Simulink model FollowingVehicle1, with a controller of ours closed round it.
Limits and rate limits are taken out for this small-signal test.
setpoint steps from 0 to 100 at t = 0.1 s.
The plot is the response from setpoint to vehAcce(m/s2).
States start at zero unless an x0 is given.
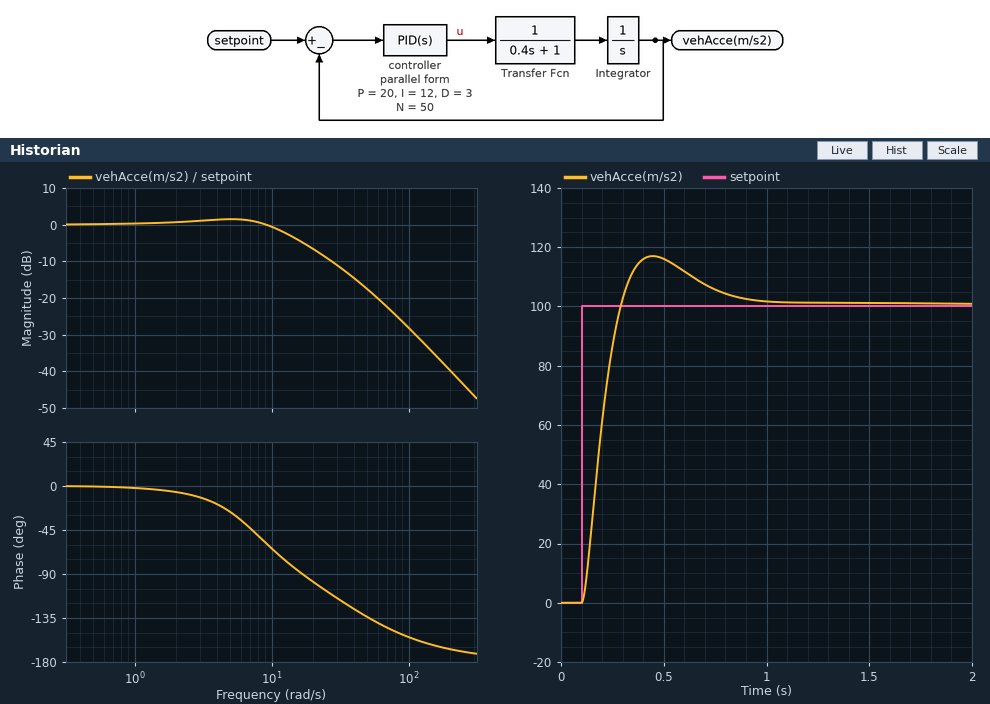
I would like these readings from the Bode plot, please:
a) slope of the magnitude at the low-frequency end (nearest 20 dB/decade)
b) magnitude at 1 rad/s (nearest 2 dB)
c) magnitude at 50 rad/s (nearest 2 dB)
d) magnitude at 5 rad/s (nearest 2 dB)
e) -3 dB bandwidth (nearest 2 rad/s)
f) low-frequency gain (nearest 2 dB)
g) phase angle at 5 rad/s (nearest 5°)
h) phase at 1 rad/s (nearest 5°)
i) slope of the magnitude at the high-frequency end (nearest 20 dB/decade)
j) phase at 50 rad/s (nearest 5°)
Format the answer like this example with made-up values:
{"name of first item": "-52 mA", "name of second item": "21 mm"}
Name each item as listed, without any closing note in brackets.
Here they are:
{"slope of the magnitude at the low-frequency end": "0 dB/decade", "magnitude at 1 rad/s": "0 dB", "magnitude at 50 rad/s": "-18 dB", "magnitude at 5 rad/s": "2 dB", "-3 dB bandwidth": "14 rad/s", "low-frequency gain": "0 dB", "phase angle at 5 rad/s": "-25°", "phase at 1 rad/s": "0°", "slope of the magnitude at the high-frequency end": "-40 dB/decade", "phase at 50 rad/s": "-135°"}
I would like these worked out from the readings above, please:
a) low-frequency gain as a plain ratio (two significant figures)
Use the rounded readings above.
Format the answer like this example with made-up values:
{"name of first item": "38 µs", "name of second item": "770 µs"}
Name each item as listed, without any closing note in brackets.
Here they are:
{"low-frequency gain as a plain ratio": "1.0"}
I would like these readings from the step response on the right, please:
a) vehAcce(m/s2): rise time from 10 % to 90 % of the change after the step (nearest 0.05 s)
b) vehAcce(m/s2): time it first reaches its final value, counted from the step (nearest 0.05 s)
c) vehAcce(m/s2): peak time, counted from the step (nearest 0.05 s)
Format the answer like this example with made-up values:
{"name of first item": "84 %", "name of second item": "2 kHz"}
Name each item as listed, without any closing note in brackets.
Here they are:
{"vehAcce(m/s2): rise time from 10 % to 90 % of the change after the step": "0.15 s", "vehAcce(m/s2): time it first reaches its final value, counted from the step": "0.20 s", "vehAcce(m/s2): peak time, counted from the step": "0.35 s"}
